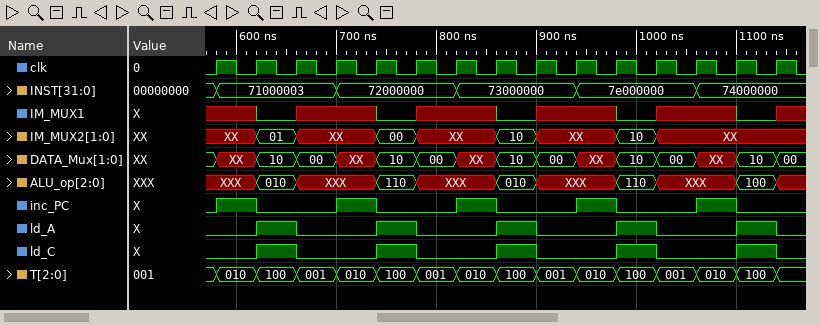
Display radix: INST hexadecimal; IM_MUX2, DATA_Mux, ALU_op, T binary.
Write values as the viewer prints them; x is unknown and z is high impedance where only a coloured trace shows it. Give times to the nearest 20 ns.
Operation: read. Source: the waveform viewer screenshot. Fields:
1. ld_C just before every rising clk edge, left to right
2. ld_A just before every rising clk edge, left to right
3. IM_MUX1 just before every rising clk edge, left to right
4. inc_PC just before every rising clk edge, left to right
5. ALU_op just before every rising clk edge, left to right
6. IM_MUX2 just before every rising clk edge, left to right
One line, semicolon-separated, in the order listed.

0 0 1 0 0 1 0 0 1 0 0 1 0 0 1; 0 0 1 0 0 1 0 0 1 0 0 1 0 0 1; x x 0 x x 0 x x 0 x x 0 x x 0; 0 1 0 0 1 0 0 1 0 0 1 0 0 1 0; XXX, XXX, 010, XXX, XXX, 110, XXX, XXX, 010, XXX, XXX, 110, XXX, XXX, 100; XX, XX, 01, XX, XX, 00, XX, XX, 10, XX, XX, 10, XX, XX, XX
